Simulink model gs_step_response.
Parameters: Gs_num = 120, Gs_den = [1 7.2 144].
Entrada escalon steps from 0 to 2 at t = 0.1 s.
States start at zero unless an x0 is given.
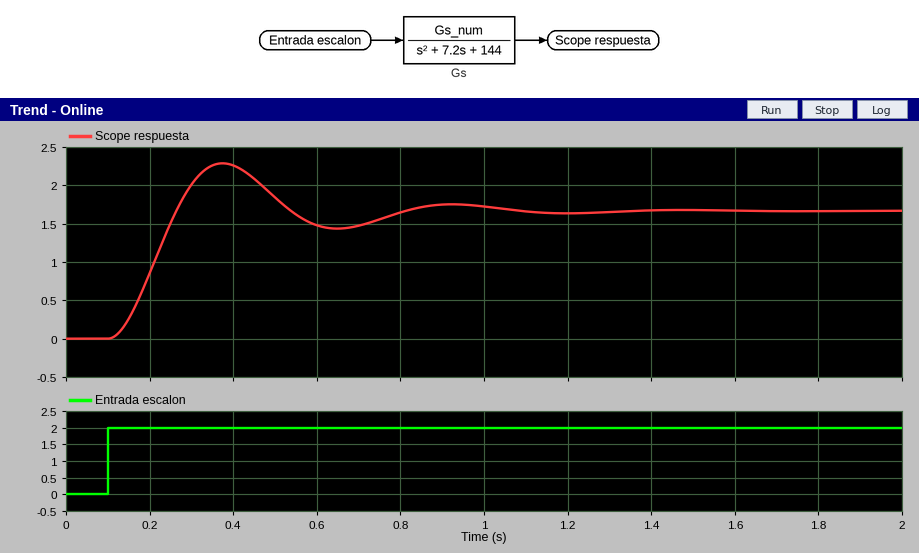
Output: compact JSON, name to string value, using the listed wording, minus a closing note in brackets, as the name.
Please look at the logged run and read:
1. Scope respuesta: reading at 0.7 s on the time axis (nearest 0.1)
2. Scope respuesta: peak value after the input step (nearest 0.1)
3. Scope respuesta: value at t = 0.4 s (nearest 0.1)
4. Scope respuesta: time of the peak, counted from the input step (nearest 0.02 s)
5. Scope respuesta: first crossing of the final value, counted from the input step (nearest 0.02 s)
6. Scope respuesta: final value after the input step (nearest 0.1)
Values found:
{"Scope respuesta: reading at 0.7 s on the time axis": "1.5", "Scope respuesta: peak value after the input step": "2.3", "Scope respuesta: value at t = 0.4 s": "2.3", "Scope respuesta: time of the peak, counted from the input step": "0.28 s", "Scope respuesta: first crossing of the final value, counted from the input step": "0.16 s", "Scope respuesta: final value after the input step": "1.7"}
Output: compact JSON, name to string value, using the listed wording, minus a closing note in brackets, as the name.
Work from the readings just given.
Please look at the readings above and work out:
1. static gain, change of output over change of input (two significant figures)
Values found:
{"static gain, change of output over change of input": "0.85"}
